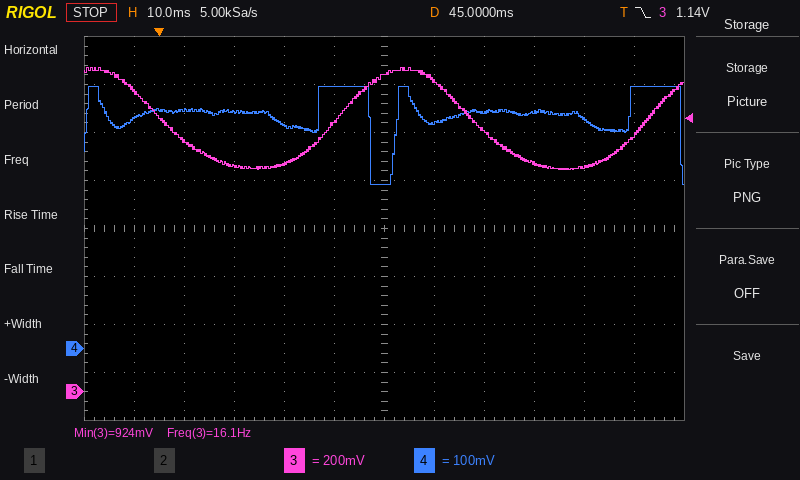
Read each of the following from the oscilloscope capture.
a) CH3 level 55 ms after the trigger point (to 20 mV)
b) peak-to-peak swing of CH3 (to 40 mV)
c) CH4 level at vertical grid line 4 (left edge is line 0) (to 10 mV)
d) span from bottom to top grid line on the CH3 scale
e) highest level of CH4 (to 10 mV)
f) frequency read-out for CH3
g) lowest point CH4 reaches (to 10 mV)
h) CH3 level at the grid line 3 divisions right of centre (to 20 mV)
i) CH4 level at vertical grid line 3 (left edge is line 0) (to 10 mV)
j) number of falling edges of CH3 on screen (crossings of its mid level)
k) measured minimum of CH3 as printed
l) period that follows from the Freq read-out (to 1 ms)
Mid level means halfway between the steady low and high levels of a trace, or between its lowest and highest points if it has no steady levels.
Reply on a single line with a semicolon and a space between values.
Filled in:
1.30 V; 440 mV; 460 mV; 1.6 V; 550 mV; 16.1 Hz; 340 mV; 960 mV; 490 mV; 2; 924 mV; 62 ms
